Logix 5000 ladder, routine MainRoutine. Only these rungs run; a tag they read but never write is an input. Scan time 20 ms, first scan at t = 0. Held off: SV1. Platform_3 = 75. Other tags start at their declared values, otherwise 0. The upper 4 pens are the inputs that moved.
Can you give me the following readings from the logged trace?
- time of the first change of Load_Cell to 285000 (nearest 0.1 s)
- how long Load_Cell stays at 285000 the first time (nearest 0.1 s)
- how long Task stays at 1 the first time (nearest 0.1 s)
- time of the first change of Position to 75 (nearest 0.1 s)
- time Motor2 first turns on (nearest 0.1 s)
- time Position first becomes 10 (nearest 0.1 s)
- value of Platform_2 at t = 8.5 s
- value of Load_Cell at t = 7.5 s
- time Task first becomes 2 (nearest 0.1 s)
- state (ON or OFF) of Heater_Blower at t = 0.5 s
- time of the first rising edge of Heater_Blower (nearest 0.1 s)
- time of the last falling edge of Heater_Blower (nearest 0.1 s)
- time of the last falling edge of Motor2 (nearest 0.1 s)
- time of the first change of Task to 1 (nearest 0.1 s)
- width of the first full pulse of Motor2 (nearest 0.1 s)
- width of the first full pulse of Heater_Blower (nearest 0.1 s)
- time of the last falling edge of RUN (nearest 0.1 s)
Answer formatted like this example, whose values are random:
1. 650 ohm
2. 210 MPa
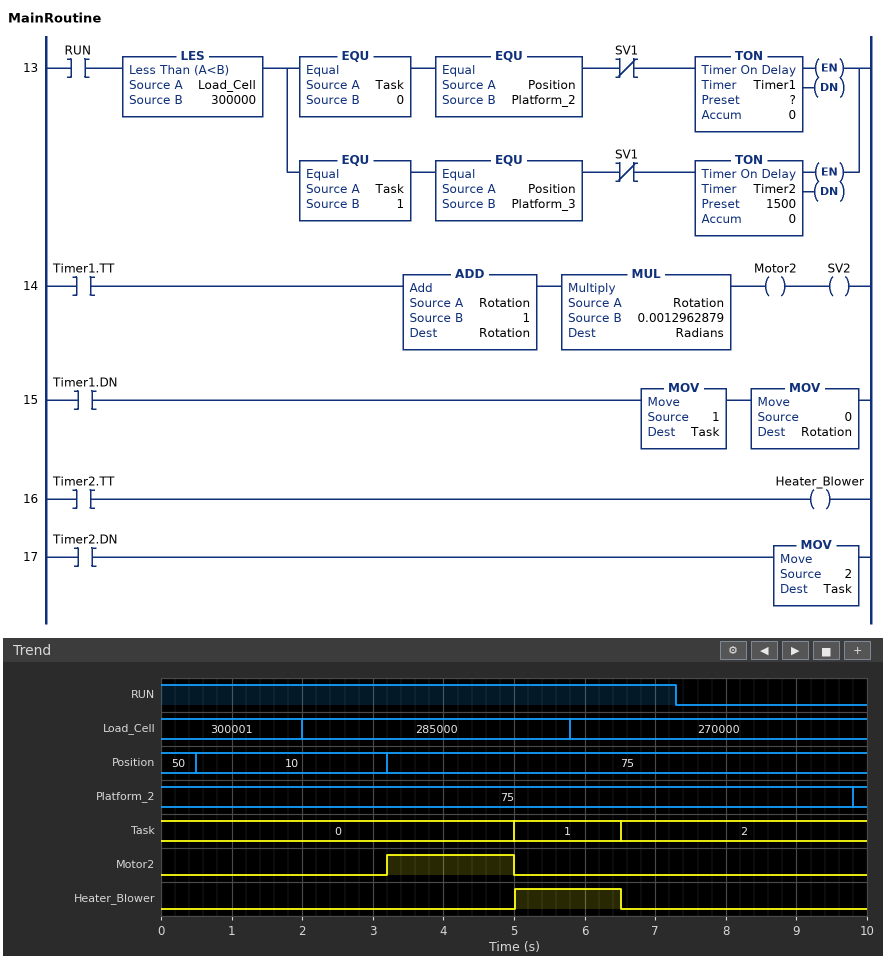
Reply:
1. 2.0 s
2. 3.8 s
3. 1.5 s
4. 3.2 s
5. 3.2 s
6. 0.5 s
7. 75
8. 270000
9. 6.5 s
10. OFF
11. 5.0 s
12. 6.5 s
13. 5.0 s
14. 5.0 s
15. 1.8 s
16. 1.5 s
17. 7.3 s
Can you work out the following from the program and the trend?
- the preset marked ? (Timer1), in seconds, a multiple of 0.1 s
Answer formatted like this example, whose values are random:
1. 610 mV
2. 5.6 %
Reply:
1. 1.8 s
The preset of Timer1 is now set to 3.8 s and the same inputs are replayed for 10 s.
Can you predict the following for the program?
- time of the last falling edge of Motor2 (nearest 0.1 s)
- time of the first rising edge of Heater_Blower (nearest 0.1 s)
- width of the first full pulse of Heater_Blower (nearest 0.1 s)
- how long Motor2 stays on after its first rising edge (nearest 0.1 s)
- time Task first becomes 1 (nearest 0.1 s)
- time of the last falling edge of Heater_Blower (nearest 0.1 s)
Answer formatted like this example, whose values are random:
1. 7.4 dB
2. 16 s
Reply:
1. 7.0 s
2. 7.0 s
3. 0.3 s
4. 3.8 s
5. 7.0 s
6. 7.3 s
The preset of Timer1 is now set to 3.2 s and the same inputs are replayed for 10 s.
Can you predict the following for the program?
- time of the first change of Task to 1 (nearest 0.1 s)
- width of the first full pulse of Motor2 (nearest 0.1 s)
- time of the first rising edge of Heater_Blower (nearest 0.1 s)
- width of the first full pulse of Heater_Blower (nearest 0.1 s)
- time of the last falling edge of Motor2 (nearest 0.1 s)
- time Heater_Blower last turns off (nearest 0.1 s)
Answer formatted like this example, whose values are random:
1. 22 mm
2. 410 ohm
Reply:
1. 6.4 s
2. 3.2 s
3. 6.4 s
4. 0.9 s
5. 6.4 s
6. 7.3 s
